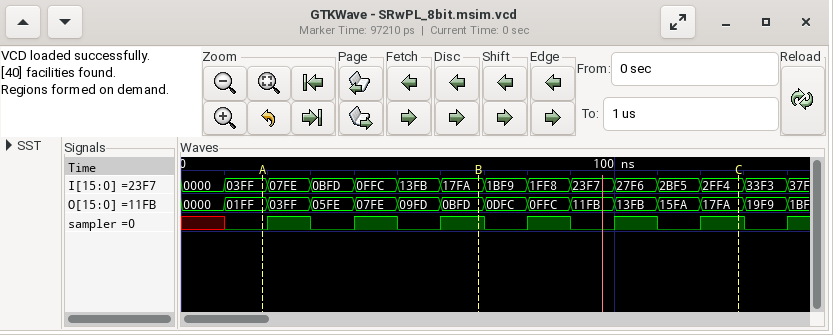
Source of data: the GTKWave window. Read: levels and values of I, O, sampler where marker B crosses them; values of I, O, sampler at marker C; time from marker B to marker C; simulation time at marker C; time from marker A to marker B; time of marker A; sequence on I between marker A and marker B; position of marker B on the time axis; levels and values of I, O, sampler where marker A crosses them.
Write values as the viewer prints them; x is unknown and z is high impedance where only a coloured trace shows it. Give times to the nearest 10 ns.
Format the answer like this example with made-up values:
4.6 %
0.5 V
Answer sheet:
I=17FA, O=0BFD, sampler=1
I=2FF4, O=17FA, sampler=1
60 ns
130 ns
50 ns
20 ns
03FF, 07FE, 0BFD, 0FFC, 13FB, 17FA
70 ns
I=03FF, O=01FF, sampler=0
